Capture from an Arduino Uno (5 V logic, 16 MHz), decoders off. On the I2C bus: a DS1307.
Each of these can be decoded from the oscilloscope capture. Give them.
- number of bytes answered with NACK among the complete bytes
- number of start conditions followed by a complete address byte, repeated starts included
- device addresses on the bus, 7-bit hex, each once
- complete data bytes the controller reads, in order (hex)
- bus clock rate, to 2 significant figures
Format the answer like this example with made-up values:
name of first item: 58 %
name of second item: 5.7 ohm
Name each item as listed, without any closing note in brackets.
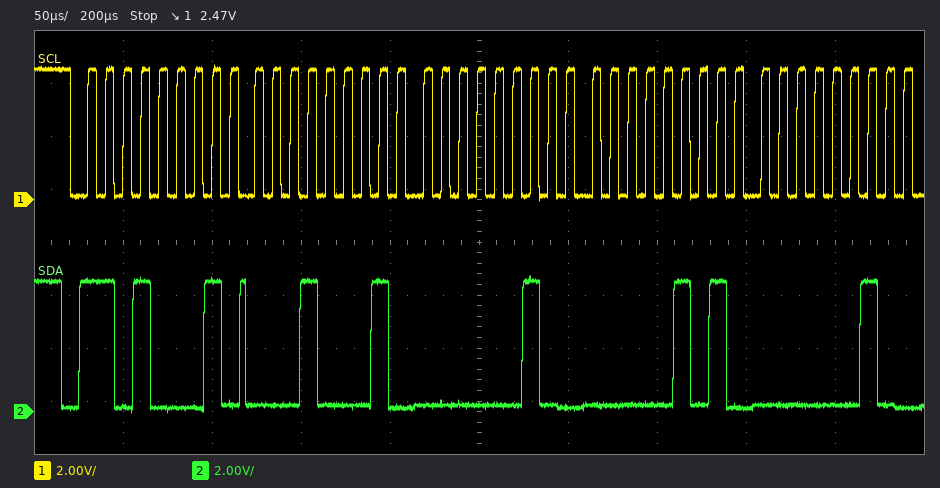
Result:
number of bytes answered with NACK among the complete bytes: 0
number of start conditions followed by a complete address byte, repeated starts included: 1
device addresses on the bus, 7-bit hex, each once: 0x68
complete data bytes the controller reads, in order: 11 02 05 02
bus clock rate, to 2 significant figures: 100 kHz
